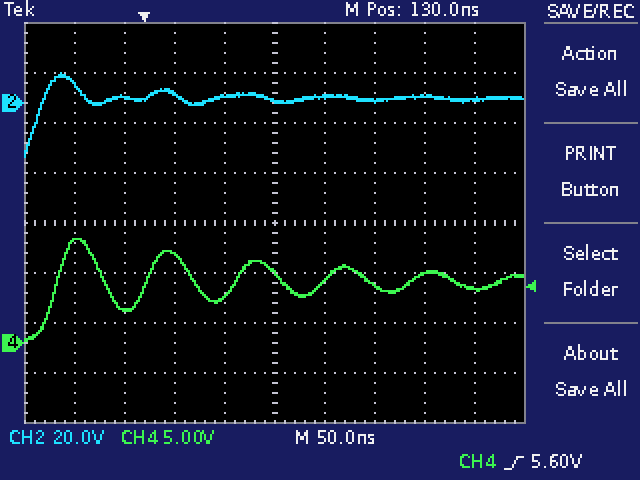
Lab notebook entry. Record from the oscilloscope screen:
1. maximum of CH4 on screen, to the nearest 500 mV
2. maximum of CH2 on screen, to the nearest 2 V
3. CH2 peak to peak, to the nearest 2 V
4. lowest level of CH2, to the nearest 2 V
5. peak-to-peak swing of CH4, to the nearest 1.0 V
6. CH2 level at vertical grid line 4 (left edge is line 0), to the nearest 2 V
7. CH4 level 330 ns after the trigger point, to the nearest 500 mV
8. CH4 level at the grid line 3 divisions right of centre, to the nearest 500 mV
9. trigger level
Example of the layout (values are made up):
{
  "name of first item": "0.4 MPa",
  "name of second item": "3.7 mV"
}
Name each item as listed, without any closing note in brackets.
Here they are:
{
  "maximum of CH4 on screen, to the nearest 500 mV": "10.5 V",
  "maximum of CH2 on screen, to the nearest 2 V": "12 V",
  "CH2 peak to peak, to the nearest 2 V": "34 V",
  "lowest level of CH2, to the nearest 2 V": "-22 V",
  "peak-to-peak swing of CH4, to the nearest 1.0 V": "10.0 V",
  "CH2 level at vertical grid line 4 (left edge is line 0), to the nearest 2 V": "2 V",
  "CH4 level 330 ns after the trigger point, to the nearest 500 mV": "5.5 V",
  "CH4 level at the grid line 3 divisions right of centre, to the nearest 500 mV": "7.0 V",
  "trigger level": "5.60 V"
}
